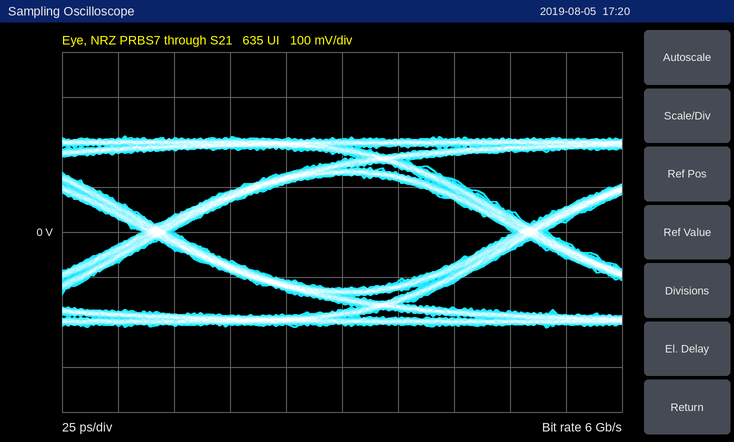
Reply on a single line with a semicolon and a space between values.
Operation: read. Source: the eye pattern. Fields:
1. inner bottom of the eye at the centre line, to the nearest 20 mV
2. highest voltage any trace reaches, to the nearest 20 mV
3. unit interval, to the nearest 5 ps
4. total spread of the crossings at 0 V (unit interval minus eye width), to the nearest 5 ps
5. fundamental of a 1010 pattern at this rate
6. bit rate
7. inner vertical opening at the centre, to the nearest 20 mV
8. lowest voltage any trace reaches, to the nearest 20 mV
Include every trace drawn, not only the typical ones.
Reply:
-120 mV; 220 mV; 165 ps; 15 ps; 3 GHz; 6 Gb/s; 260 mV; -220 mV
